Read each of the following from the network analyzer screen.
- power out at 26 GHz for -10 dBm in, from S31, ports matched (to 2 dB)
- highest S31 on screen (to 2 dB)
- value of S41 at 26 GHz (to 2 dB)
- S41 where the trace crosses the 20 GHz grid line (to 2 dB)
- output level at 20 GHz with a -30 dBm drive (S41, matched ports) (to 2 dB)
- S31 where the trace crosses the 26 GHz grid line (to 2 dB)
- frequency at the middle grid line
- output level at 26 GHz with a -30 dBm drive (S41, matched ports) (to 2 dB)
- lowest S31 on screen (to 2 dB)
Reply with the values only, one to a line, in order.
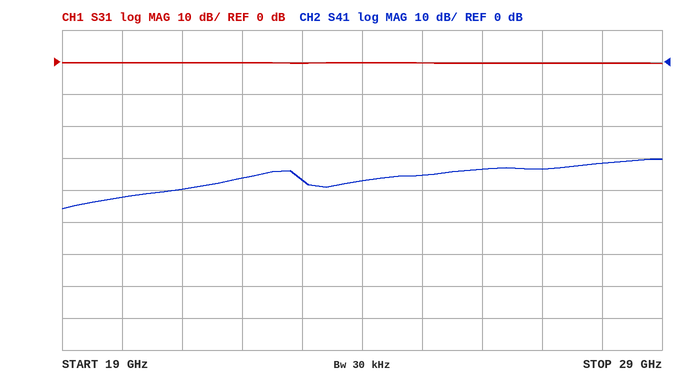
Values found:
-10 dBm
0 dB
-34 dB
-42 dB
-72 dBm
0 dB
24 GHz
-64 dBm
0 dB
